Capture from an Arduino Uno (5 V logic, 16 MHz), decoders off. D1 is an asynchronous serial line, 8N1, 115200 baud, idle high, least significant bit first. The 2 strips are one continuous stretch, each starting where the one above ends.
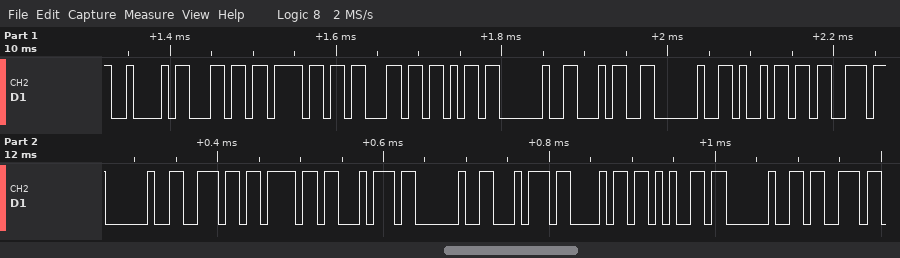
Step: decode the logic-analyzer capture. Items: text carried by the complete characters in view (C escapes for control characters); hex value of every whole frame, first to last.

"Block 4 is not the s"
42 6C 6F 63 6B 20 34 20 69 73 20 6E 6F 74 20 74 68 65 20 73
